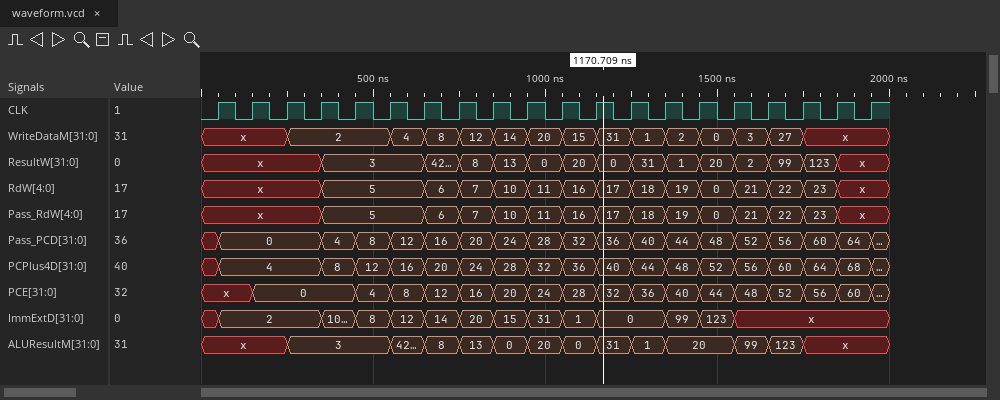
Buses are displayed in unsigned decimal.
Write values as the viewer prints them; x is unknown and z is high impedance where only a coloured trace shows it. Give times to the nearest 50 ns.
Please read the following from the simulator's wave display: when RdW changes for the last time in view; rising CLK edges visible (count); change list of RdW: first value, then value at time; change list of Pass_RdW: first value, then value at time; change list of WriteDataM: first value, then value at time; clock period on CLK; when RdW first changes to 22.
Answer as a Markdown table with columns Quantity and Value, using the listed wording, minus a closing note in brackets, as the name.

| Quantity | Value |
|---|---|
| when RdW changes for the last time in view | 1850 ns |
| rising CLK edges visible | 20 |
| change list of RdW: first value, then value at time | x, 5 at 350 ns, 6 at 650 ns, 7 at 750 ns, 10 at 850 ns, 11 at 950 ns, 16 at 1050 ns, 17 at 1150 ns, 18 at 1250 ns, 19 at 1350 ns, 0 at 1450 ns, 21 at 1550 ns, 22 at 1650 ns, 23 at 1750 ns, x at 1850 ns |
| change list of Pass_RdW: first value, then value at time | x, 5 at 350 ns, 6 at 650 ns, 7 at 750 ns, 10 at 850 ns, 11 at 950 ns, 16 at 1050 ns, 17 at 1150 ns, 18 at 1250 ns, 19 at 1350 ns, 0 at 1450 ns, 21 at 1550 ns, 22 at 1650 ns, 23 at 1750 ns, x at 1850 ns |
| change list of WriteDataM: first value, then value at time | x, 2 at 250 ns, 4 at 550 ns, 8 at 650 ns, 12 at 750 ns, 14 at 850 ns, 20 at 950 ns, 15 at 1050 ns, 31 at 1150 ns, 1 at 1250 ns, 2 at 1350 ns, 0 at 1450 ns, 3 at 1550 ns, 27 at 1650 ns, x at 1750 ns |
| clock period on CLK | 100 ns |
| when RdW first changes to 22 | 1650 ns |
